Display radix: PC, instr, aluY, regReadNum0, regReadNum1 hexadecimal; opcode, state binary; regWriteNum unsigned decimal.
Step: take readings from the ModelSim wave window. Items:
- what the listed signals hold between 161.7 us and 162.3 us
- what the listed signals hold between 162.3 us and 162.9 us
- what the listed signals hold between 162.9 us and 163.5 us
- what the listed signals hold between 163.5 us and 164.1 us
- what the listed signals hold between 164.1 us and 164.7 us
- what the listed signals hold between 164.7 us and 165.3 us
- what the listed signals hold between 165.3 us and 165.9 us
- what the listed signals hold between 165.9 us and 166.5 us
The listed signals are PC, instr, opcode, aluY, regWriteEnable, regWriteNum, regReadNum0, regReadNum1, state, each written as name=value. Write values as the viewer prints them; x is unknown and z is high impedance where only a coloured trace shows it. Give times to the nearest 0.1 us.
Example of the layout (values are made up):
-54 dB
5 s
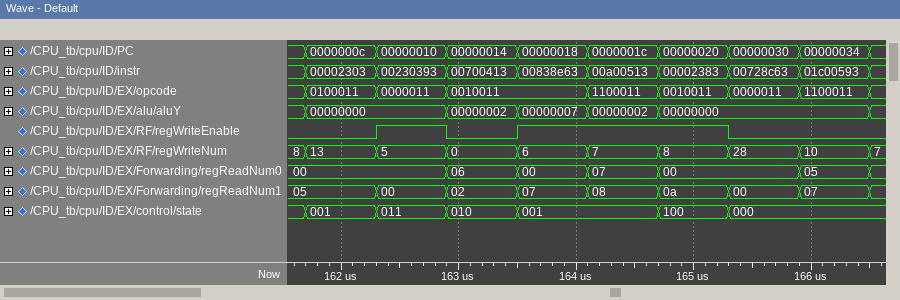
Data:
PC=0000000c, instr=00002303, opcode=0100011, aluY=00000000, regWriteEnable=0, regWriteNum=13, regReadNum0=00, regReadNum1=05, state=001
PC=00000010, instr=00230393, opcode=0000011, aluY=00000000, regWriteEnable=1, regWriteNum=5, regReadNum0=00, regReadNum1=00, state=011
PC=00000014, instr=00700413, opcode=0010011, aluY=00000002, regWriteEnable=0, regWriteNum=0, regReadNum0=06, regReadNum1=02, state=010
PC=00000018, instr=00838e63, opcode=0010011, aluY=00000007, regWriteEnable=1, regWriteNum=6, regReadNum0=00, regReadNum1=07, state=001
PC=0000001c, instr=00a00513, opcode=1100011, aluY=00000002, regWriteEnable=1, regWriteNum=7, regReadNum0=07, regReadNum1=08, state=001
PC=00000020, instr=00002383, opcode=0010011, aluY=00000000, regWriteEnable=1, regWriteNum=8, regReadNum0=00, regReadNum1=0a, state=100
PC=00000030, instr=00728c63, opcode=0000011, aluY=00000000, regWriteEnable=0, regWriteNum=28, regReadNum0=00, regReadNum1=00, state=000
PC=00000034, instr=01c00593, opcode=1100011, aluY=00000000, regWriteEnable=0, regWriteNum=10, regReadNum0=05, regReadNum1=07, state=000
